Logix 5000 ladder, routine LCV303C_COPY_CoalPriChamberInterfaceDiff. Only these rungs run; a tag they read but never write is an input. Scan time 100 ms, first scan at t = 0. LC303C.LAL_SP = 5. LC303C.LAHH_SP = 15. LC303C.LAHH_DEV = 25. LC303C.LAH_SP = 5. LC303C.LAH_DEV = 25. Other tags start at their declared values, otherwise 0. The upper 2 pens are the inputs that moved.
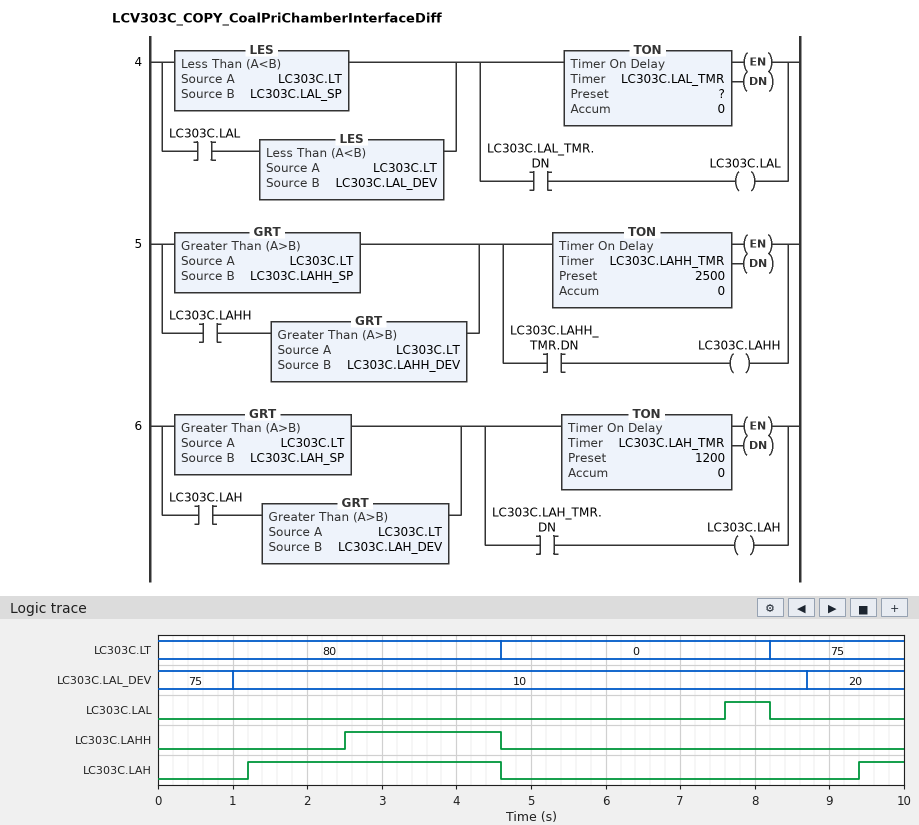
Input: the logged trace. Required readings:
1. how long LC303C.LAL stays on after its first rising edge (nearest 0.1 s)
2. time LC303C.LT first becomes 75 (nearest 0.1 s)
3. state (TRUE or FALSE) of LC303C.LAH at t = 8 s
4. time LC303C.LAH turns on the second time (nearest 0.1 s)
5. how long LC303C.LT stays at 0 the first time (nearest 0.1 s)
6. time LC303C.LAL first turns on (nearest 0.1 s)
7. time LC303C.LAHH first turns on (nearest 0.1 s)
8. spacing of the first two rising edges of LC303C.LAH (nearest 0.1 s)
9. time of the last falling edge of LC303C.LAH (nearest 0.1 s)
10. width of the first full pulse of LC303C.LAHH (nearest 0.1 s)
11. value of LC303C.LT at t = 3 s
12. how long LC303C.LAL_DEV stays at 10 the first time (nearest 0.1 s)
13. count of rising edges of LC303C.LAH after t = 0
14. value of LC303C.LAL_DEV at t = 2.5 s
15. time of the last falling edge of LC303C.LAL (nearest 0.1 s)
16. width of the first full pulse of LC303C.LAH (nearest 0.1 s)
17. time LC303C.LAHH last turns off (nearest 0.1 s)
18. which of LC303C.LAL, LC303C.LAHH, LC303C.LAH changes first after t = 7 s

0.6 s
8.2 s
FALSE
9.4 s
3.6 s
7.6 s
2.5 s
8.2 s
4.6 s
2.1 s
80
7.7 s
2
10
8.2 s
3.4 s
4.6 s
LC303C.LAL
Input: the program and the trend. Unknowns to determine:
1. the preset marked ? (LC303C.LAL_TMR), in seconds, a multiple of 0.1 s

3.0 s
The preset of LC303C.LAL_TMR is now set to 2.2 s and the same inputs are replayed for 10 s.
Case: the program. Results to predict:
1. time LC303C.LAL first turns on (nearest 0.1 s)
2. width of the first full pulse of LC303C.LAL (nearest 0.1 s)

6.8 s
1.4 s
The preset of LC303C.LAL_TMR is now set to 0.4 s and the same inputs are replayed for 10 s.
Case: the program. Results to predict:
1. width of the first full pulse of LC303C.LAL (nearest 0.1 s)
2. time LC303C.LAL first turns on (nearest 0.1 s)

3.2 s
5.0 s
